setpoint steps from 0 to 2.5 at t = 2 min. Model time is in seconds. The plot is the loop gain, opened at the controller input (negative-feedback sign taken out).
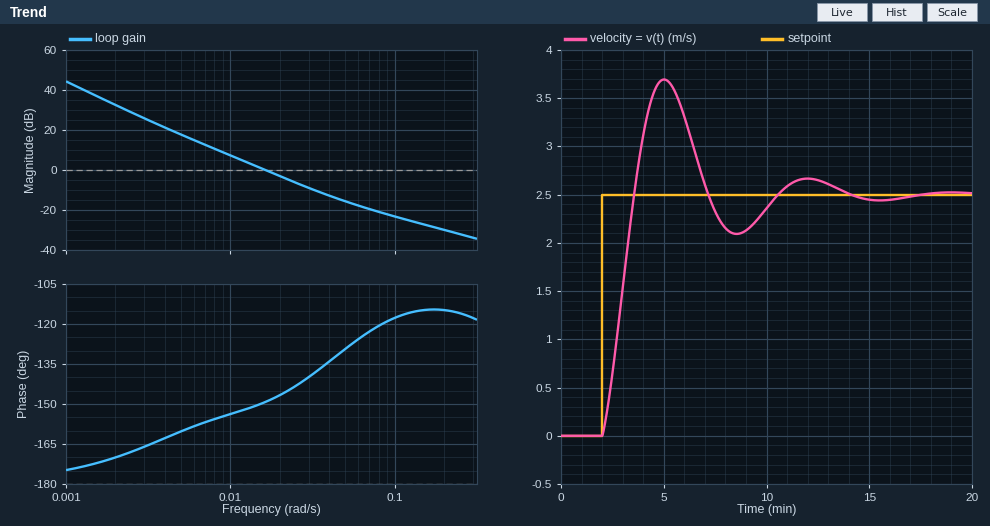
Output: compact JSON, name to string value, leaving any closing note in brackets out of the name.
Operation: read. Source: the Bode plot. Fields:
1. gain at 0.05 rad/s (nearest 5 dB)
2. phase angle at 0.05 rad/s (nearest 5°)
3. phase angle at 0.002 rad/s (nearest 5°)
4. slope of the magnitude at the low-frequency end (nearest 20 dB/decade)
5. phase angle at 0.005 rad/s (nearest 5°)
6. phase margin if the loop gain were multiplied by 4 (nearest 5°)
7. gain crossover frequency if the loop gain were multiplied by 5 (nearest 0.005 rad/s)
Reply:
{"gain at 0.05 rad/s": "-15 dB", "phase angle at 0.05 rad/s": "-130°", "phase angle at 0.002 rad/s": "-170°", "slope of the magnitude at the low-frequency end": "-40 dB/decade", "phase angle at 0.005 rad/s": "-160°", "phase margin if the loop gain were multiplied by 4": "45°", "gain crossover frequency if the loop gain were multiplied by 5": "0.045 rad/s"}
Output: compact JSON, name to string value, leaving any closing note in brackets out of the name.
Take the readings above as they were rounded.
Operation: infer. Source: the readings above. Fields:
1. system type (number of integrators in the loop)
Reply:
{"system type": "2"}
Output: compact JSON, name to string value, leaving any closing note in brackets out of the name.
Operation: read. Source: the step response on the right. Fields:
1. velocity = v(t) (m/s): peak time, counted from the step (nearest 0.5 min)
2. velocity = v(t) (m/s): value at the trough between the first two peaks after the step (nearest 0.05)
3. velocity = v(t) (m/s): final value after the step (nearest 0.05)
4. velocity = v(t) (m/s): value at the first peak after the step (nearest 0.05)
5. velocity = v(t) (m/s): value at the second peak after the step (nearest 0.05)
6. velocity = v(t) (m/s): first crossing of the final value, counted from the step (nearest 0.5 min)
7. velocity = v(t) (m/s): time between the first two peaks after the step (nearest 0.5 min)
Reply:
{"velocity = v(t) (m/s): peak time, counted from the step": "3.0 min", "velocity = v(t) (m/s): value at the trough between the first two peaks after the step": "2.10", "velocity = v(t) (m/s): final value after the step": "2.50", "velocity = v(t) (m/s): value at the first peak after the step": "3.70", "velocity = v(t) (m/s): value at the second peak after the step": "2.65", "velocity = v(t) (m/s): first crossing of the final value, counted from the step": "1.5 min", "velocity = v(t) (m/s): time between the first two peaks after the step": "7.0 min"}
